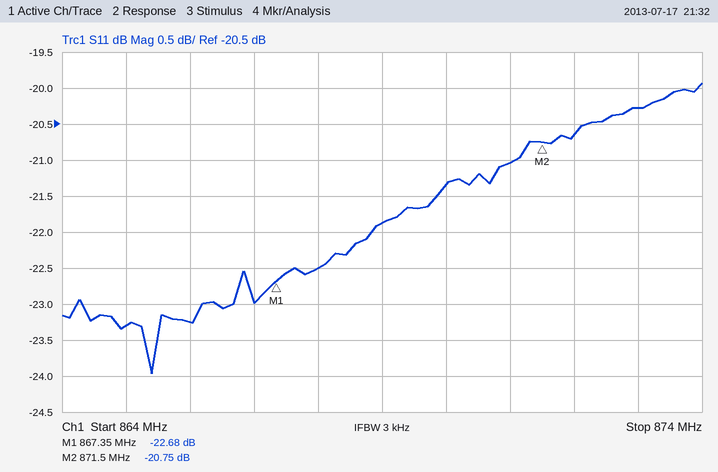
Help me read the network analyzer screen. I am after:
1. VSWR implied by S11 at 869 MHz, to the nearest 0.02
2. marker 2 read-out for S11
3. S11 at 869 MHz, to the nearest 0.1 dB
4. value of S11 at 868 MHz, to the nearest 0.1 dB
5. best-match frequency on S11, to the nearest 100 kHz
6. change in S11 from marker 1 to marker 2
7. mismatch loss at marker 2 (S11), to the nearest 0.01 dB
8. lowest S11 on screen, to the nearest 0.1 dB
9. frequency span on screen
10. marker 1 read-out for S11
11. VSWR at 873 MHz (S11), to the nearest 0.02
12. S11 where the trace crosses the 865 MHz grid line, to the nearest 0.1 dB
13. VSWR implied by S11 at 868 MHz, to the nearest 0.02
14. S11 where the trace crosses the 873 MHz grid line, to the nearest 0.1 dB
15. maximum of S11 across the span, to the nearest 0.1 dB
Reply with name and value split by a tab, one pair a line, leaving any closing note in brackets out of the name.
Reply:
VSWR implied by S11 at 869 MHz, to the nearest 0.02	1.18
marker 2 read-out for S11	-20.75 dB
S11 at 869 MHz, to the nearest 0.1 dB	-21.9 dB
value of S11 at 868 MHz, to the nearest 0.1 dB	-22.5 dB
best-match frequency on S11, to the nearest 100 kHz	865.4 MHz
change in S11 from marker 1 to marker 2	1.93 dB
mismatch loss at marker 2 (S11), to the nearest 0.01 dB	0.04 dB
lowest S11 on screen, to the nearest 0.1 dB	-24.0 dB
frequency span on screen	10 MHz
marker 1 read-out for S11	-22.68 dB
VSWR at 873 MHz (S11), to the nearest 0.02	1.22
S11 where the trace crosses the 865 MHz grid line, to the nearest 0.1 dB	-23.3 dB
VSWR implied by S11 at 868 MHz, to the nearest 0.02	1.16
S11 where the trace crosses the 873 MHz grid line, to the nearest 0.1 dB	-20.3 dB
maximum of S11 across the span, to the nearest 0.1 dB	-19.9 dB
